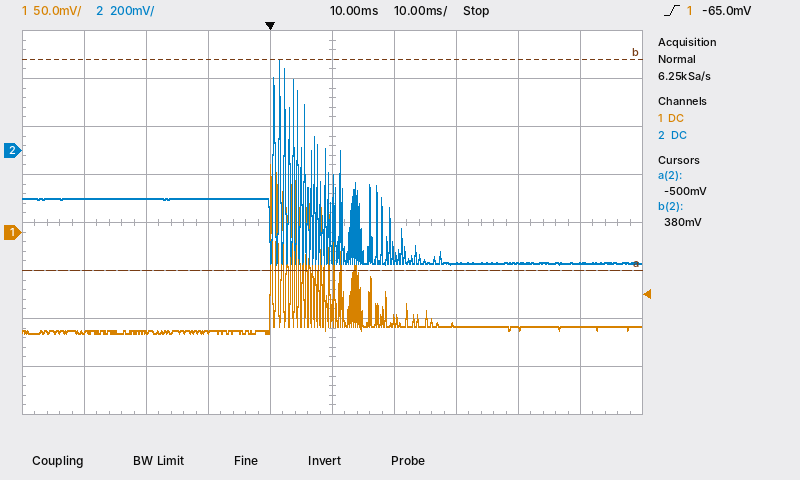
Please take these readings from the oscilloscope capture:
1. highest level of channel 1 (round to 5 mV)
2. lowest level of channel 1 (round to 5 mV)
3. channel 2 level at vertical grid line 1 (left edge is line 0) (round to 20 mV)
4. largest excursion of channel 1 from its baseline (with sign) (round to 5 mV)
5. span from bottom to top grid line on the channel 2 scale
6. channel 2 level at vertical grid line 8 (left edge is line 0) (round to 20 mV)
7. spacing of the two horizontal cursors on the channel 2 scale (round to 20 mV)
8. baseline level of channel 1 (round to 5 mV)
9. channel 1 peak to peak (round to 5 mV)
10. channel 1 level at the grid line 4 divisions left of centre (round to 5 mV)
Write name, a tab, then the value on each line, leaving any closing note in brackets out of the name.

highest level of channel 1	70 mV
lowest level of channel 1	-105 mV
channel 2 level at vertical grid line 1 (left edge is line 0)	-200 mV
largest excursion of channel 1 from its baseline (with sign)	+170 mV
span from bottom to top grid line on the channel 2 scale	1.6 V
channel 2 level at vertical grid line 8 (left edge is line 0)	-460 mV
spacing of the two horizontal cursors on the channel 2 scale	880 mV
baseline level of channel 1	-100 mV
channel 1 peak to peak	175 mV
channel 1 level at the grid line 4 divisions left of centre	-105 mV
